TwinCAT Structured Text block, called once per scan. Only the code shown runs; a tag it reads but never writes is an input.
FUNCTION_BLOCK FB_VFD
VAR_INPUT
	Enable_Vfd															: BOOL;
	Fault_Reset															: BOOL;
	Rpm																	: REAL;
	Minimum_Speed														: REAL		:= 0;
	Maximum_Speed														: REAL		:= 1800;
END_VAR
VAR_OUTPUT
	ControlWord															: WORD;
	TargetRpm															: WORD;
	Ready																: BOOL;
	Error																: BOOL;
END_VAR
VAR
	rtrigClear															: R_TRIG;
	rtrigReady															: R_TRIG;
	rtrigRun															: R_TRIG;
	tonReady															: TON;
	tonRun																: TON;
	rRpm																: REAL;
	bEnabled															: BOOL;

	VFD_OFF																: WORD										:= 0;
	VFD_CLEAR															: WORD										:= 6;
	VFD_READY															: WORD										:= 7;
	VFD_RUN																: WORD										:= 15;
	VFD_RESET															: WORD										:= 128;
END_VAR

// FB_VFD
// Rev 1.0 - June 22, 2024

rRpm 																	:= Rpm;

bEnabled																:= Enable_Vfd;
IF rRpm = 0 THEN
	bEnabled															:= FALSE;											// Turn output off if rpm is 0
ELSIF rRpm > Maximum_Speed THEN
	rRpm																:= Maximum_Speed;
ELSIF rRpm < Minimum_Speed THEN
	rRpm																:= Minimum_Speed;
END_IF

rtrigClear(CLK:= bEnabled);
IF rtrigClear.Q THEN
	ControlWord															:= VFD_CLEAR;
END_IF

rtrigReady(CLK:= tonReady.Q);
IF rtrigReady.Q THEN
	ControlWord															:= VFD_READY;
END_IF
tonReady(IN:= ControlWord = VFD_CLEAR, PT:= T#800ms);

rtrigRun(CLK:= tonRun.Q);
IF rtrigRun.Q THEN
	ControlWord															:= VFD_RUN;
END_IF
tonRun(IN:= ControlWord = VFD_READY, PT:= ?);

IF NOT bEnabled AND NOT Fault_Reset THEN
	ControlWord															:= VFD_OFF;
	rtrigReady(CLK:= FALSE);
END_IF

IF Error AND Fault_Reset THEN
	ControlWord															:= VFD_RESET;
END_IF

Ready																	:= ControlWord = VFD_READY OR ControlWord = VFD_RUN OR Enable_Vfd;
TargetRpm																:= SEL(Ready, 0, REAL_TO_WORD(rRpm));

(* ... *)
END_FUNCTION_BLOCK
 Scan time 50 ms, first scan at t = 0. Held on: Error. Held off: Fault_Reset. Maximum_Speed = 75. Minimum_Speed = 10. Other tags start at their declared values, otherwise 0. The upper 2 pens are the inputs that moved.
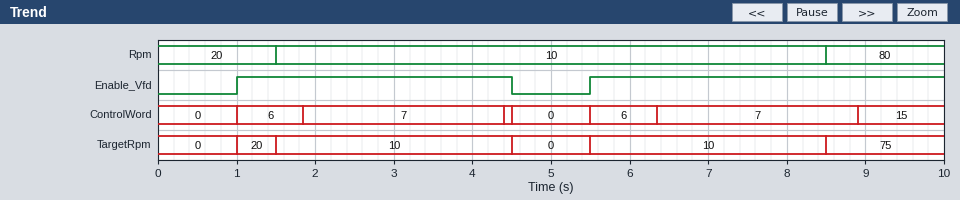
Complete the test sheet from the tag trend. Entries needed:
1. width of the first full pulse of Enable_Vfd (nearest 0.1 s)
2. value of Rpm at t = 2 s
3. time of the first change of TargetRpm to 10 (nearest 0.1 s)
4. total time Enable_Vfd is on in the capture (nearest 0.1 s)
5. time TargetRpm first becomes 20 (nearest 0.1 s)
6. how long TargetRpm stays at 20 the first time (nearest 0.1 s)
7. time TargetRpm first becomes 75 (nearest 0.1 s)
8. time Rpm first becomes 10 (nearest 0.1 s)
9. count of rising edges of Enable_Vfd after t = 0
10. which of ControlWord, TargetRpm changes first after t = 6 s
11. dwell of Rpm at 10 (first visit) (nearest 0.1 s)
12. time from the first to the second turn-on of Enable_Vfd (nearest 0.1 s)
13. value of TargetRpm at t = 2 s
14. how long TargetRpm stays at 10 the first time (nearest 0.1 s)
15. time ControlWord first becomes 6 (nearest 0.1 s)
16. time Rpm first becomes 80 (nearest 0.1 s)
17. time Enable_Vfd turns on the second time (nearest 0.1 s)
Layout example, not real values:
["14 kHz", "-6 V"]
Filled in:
["3.5 s", "10", "1.5 s", "8.0 s", "1.0 s", "0.5 s", "8.5 s", "1.5 s", "2", "ControlWord", "7.0 s", "4.5 s", "10", "3.0 s", "1.0 s", "8.5 s", "5.5 s"]
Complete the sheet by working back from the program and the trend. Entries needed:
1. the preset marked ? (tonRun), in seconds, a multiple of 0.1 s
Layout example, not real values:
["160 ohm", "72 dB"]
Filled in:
["2.5 s"]
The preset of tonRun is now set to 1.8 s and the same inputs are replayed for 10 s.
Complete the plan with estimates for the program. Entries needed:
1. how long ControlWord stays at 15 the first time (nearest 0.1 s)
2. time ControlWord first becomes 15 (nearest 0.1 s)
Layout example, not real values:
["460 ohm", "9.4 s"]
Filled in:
["0.8 s", "3.7 s"]
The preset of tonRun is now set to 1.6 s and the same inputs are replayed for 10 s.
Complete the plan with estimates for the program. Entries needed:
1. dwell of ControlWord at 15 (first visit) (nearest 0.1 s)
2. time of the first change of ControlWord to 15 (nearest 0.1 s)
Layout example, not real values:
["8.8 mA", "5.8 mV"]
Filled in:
["1.0 s", "3.5 s"]
